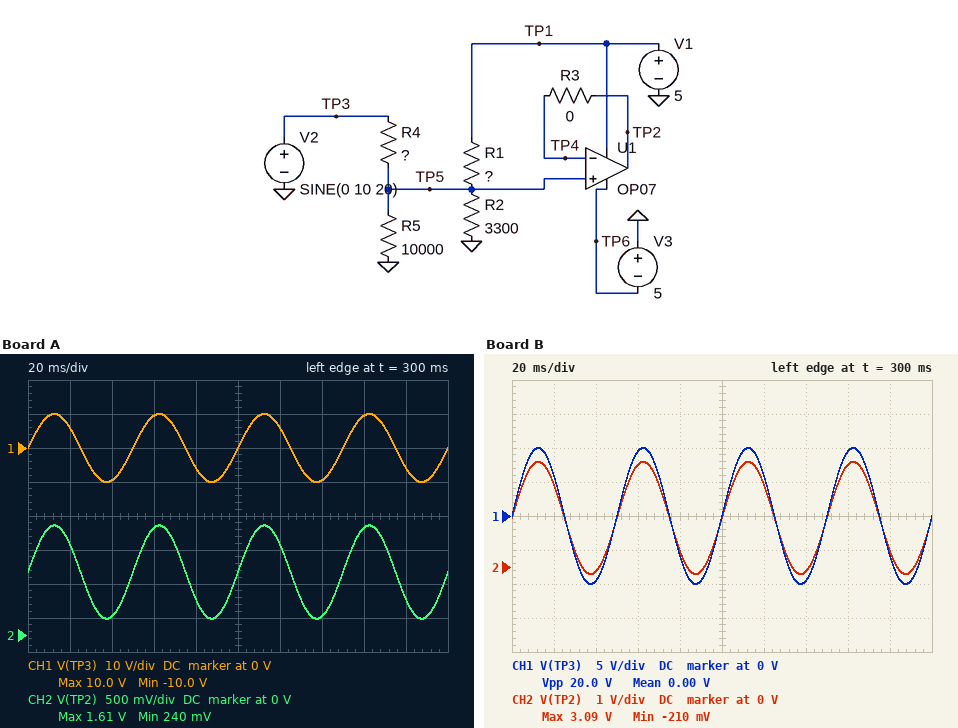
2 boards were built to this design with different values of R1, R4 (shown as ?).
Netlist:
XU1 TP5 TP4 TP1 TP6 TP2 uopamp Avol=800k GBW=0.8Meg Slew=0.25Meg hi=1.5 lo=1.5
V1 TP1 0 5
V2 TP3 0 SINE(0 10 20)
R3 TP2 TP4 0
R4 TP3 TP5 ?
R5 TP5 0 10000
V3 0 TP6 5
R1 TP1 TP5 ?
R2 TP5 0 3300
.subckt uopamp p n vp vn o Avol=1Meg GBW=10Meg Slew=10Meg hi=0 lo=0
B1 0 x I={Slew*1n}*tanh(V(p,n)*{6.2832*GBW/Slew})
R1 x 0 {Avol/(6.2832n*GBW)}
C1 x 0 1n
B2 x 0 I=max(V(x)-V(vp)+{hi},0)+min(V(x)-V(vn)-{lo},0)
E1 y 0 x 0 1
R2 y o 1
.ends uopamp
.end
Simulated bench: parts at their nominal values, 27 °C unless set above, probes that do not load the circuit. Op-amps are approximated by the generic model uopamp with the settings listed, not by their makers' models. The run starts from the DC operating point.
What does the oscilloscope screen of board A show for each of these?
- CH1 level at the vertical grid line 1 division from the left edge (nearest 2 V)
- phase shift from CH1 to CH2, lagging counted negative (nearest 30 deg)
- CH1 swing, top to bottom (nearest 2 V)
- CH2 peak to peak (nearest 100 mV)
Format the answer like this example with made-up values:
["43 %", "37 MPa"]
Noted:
["6 V", "0 deg", "20 V", "1.4 V"]
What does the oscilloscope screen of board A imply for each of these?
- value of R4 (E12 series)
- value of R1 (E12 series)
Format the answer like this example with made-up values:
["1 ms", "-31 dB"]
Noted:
["27 kΩ", "10 kΩ"]
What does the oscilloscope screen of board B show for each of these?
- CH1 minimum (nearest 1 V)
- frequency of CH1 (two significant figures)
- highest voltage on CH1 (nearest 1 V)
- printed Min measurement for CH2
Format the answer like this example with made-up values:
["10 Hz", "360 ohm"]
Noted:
["-10 V", "20 Hz", "10 V", "-210 mV"]
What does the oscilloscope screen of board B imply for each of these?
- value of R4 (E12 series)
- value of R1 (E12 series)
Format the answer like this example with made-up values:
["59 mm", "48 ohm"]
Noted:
["8.2 kΩ", "4.7 kΩ"]
